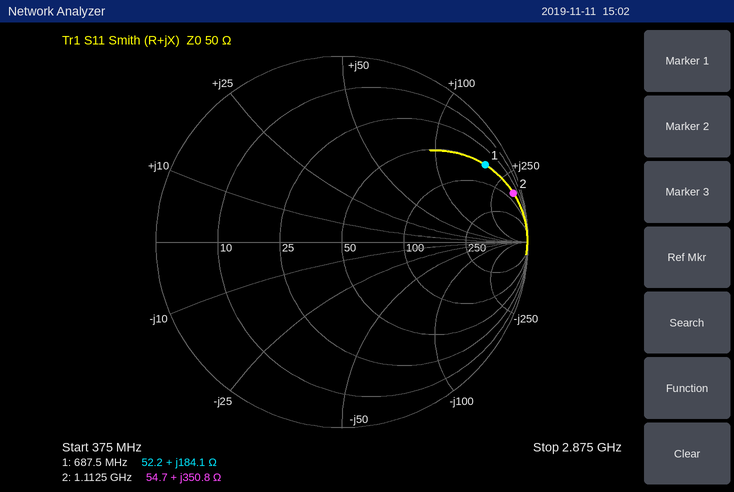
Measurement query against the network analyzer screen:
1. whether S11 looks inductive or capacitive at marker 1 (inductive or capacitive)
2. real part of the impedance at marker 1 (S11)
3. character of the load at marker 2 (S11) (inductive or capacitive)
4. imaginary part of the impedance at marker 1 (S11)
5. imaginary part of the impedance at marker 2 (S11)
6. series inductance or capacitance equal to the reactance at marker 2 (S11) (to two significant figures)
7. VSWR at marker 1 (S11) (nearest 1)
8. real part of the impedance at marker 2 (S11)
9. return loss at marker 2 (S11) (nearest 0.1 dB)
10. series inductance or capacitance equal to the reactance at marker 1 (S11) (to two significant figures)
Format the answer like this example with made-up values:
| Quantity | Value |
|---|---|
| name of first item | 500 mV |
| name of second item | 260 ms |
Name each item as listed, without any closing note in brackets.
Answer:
| Quantity | Value |
|---|---|
| whether S11 looks inductive or capacitive at marker 1 | inductive |
| real part of the impedance at marker 1 | 52.2 Ω |
| character of the load at marker 2 (S11) | inductive |
| imaginary part of the impedance at marker 1 | +184.1 Ω |
| imaginary part of the impedance at marker 2 | +350.8 Ω |
| series inductance or capacitance equal to the reactance at marker 2 (S11) | 50 nH |
| VSWR at marker 1 (S11) | 15 |
| real part of the impedance at marker 2 | 54.7 Ω |
| return loss at marker 2 (S11) | 0.4 dB |
| series inductance or capacitance equal to the reactance at marker 1 (S11) | 43 nH |
